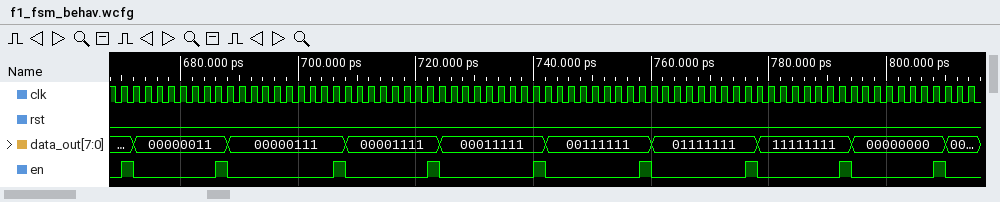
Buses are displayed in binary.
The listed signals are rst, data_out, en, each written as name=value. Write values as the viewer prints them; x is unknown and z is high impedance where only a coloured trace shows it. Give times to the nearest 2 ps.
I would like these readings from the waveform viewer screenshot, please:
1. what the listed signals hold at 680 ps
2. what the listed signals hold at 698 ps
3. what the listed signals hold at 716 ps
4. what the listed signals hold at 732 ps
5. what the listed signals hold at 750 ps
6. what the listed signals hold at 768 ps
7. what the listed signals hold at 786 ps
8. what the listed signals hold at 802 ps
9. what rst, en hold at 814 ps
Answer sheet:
rst=0, data_out=00000011, en=0
rst=0, data_out=00000111, en=0
rst=0, data_out=00001111, en=0
rst=0, data_out=00011111, en=0
rst=0, data_out=00111111, en=0
rst=0, data_out=01111111, en=0
rst=0, data_out=11111111, en=0
rst=0, data_out=00000000, en=0
rst=0, en=0
